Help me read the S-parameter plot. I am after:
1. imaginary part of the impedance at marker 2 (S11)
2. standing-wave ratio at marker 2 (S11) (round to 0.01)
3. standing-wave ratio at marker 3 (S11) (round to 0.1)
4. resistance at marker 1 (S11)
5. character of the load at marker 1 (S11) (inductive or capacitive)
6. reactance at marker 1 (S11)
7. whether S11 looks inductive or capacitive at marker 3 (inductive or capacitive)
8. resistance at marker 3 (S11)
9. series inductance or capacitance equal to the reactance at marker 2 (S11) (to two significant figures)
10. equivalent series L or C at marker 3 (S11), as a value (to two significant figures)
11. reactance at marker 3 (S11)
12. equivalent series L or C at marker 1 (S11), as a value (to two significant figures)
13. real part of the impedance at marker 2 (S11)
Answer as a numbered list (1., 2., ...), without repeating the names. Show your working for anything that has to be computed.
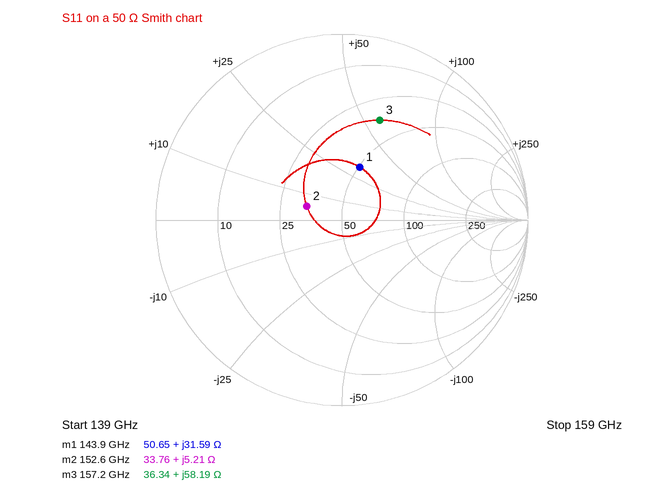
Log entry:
1. +5.21 Ω
2. 1.51
3. 3.7
4. 50.65 Ω
5. inductive
6. +31.59 Ω
7. inductive
8. 36.34 Ω
9. L = 5.21 Ω/(2π × 152.6 GHz) ≈ 5.4 pH
10. L = 58.19 Ω/(2π × 157.2 GHz) ≈ 59 pH
11. +58.19 Ω
12. L = 31.59 Ω/(2π × 143.9 GHz) ≈ 35 pH
13. 33.76 Ω
